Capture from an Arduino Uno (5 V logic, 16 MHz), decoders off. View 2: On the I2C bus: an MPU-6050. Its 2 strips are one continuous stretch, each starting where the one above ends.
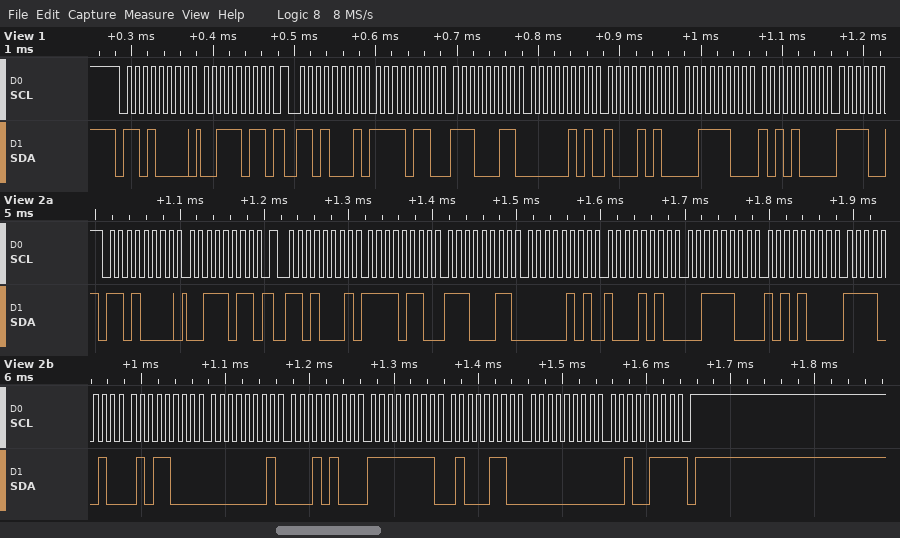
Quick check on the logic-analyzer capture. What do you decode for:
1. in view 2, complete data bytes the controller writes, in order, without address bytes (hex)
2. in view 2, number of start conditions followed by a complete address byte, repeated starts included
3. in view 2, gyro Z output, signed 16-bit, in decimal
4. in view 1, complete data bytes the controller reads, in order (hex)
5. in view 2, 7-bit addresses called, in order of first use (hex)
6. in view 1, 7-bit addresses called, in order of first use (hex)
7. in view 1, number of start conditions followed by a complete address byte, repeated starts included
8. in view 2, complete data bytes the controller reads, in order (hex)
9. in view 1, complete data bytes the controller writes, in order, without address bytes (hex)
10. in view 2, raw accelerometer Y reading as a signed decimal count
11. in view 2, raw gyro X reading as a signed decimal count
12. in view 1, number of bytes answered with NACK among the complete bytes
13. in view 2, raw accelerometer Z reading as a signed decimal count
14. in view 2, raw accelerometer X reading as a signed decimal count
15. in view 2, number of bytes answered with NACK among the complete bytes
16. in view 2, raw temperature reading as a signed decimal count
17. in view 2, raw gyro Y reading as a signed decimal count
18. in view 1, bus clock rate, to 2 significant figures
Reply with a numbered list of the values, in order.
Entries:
1. 3B
2. 2
3. 39
4. F6 E3 05 8A 3C A8
5. 0x68
6. 0x68
7. 2
8. F6 E3 05 8A 3C A8 F2 58 01 14 FF 46 00 27
9. 3B
10. 1418
11. 276
12. 0
13. 15528
14. -2333
15. 1
16. -3496
17. -186
18. 100 kHz
